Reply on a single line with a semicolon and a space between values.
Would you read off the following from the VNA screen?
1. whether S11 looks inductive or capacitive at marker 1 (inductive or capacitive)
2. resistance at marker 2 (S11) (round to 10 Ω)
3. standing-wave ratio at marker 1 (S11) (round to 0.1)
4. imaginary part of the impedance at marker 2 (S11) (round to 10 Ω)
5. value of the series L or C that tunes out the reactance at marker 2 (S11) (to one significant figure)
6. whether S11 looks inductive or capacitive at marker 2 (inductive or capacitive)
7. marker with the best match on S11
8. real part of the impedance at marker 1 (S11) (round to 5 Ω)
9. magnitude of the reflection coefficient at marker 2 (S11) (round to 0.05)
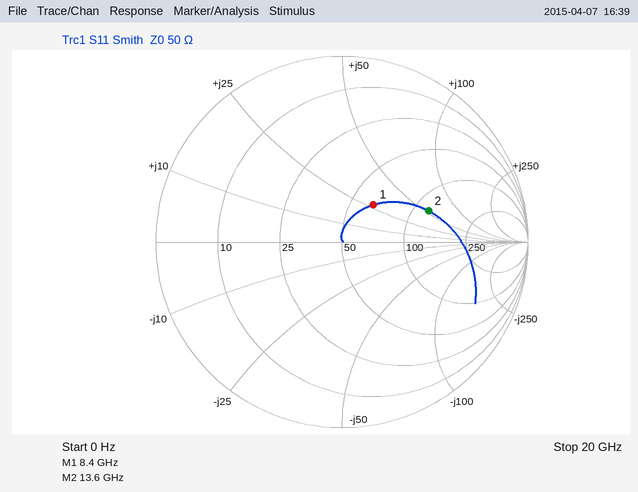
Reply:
inductive; 120 Ω; 1.7; +50 Ω; 200 fF; inductive; marker 1; 65 Ω; 0.50
